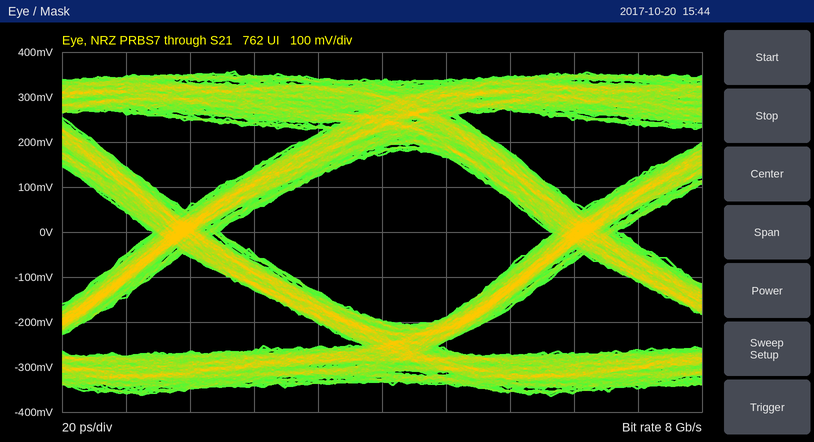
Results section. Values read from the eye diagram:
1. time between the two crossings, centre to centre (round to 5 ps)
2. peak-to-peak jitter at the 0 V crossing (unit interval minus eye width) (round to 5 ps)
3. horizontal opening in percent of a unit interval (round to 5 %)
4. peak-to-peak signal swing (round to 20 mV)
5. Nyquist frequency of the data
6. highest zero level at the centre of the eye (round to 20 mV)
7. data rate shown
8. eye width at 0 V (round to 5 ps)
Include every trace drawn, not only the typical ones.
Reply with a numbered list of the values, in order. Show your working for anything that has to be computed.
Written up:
1. 125 ps
2. 20 ps
3. 105 ps / 125 ps ≈ 84.0 %, so 85 % to the nearest 5 %
4. 720 mV
5. 4 GHz
6. -200 mV
7. 8 Gb/s
8. 105 ps
